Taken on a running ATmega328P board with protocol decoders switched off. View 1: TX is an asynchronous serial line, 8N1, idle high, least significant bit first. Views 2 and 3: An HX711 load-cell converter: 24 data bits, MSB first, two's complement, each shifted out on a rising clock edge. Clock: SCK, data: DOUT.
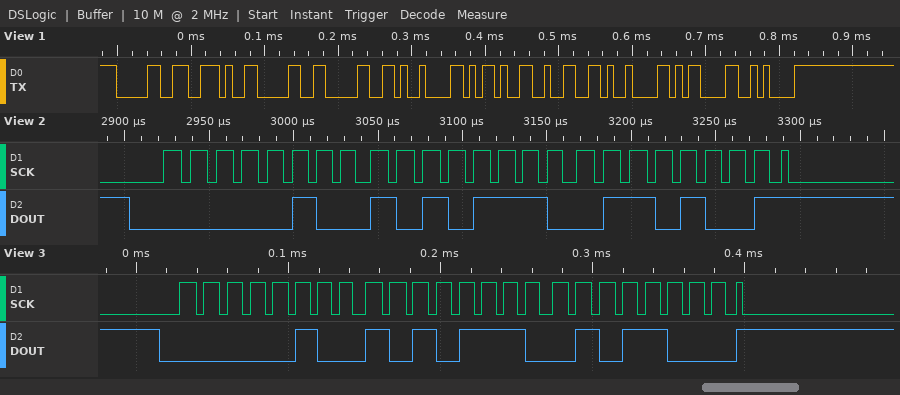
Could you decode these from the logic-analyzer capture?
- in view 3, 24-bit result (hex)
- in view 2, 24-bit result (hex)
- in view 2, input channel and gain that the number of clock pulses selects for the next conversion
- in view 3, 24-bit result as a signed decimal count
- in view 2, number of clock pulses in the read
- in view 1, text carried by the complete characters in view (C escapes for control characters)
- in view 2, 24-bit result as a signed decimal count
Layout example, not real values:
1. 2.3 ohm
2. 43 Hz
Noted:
1. 0x04AE58
2. 0x04AE69
3. channel A, gain 128
4. 306776
5. 25
6. "0.00\t-2\t\r\n"
7. 306793
